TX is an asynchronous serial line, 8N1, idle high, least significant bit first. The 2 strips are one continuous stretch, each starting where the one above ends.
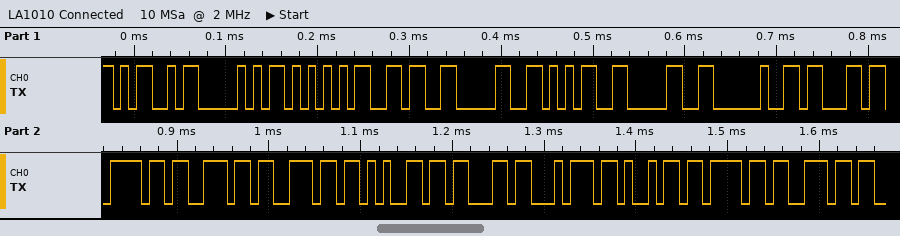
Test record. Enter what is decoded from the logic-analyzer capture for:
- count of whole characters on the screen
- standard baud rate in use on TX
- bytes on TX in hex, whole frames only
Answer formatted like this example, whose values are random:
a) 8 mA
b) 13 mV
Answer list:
a) 18
b) 115200 baud
c) 0x4D 0x50 0x55 0x36 0x30 0x35 0x30 0x20 0x63 0x6F 0x6E 0x6E 0x65 0x63 0x74 0x69 0x6F 0x6E
